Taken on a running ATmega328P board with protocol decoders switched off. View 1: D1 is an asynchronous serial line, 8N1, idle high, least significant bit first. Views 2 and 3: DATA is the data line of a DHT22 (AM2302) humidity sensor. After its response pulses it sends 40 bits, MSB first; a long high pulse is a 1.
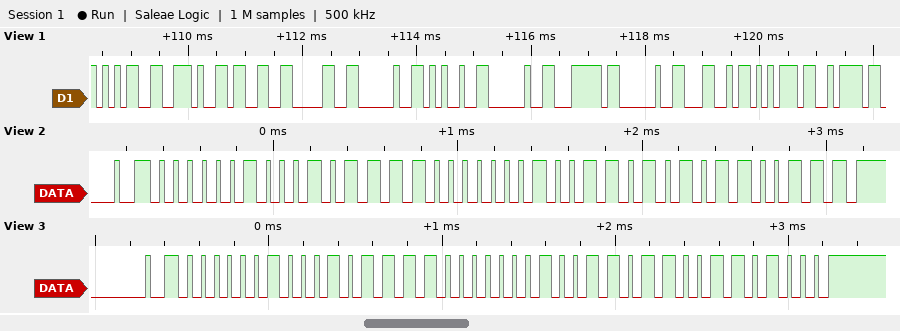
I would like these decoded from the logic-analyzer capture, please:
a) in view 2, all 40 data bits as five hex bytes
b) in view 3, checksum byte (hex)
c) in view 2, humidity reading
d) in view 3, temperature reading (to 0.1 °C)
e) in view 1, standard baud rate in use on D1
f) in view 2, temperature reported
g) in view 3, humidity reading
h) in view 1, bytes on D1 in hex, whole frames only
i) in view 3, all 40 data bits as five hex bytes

02 2F 01 35 67
0x68
55.9 %
31.0 °C
9600 baud
30.9 °C
55.9 %
35 2E 33 30 20 25 20 7C 20 4C 75 7A
02 2F 01 36 68
